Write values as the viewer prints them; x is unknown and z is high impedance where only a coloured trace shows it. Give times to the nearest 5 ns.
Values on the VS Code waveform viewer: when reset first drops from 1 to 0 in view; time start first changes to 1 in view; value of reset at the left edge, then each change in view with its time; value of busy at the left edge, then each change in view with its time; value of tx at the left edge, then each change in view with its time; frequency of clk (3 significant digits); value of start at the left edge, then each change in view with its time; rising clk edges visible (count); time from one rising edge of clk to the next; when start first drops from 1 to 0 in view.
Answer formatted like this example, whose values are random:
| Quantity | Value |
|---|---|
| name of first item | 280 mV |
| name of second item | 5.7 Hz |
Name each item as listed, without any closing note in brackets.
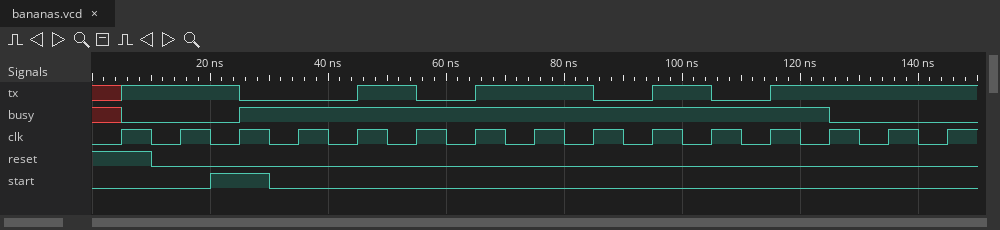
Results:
| Quantity | Value |
|---|---|
| when reset first drops from 1 to 0 in view | 10 ns |
| time start first changes to 1 in view | 20 ns |
| value of reset at the left edge, then each change in view with its time | 1, 0 at 10 ns |
| value of busy at the left edge, then each change in view with its time | x, 0 at 5 ns, 1 at 25 ns, 0 at 125 ns |
| value of tx at the left edge, then each change in view with its time | x, 1 at 5 ns, 0 at 25 ns, 1 at 45 ns, 0 at 55 ns, 1 at 65 ns, 0 at 85 ns, 1 at 95 ns, 0 at 105 ns, 1 at 115 ns |
| frequency of clk | 100 MHz |
| value of start at the left edge, then each change in view with its time | 0, 1 at 20 ns, 0 at 30 ns |
| rising clk edges visible | 15 |
| time from one rising edge of clk to the next | 10 ns |
| when start first drops from 1 to 0 in view | 30 ns |
